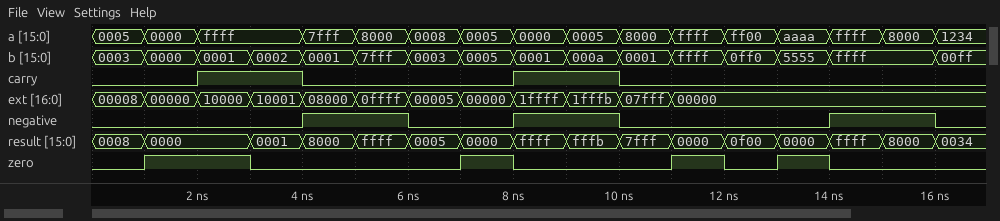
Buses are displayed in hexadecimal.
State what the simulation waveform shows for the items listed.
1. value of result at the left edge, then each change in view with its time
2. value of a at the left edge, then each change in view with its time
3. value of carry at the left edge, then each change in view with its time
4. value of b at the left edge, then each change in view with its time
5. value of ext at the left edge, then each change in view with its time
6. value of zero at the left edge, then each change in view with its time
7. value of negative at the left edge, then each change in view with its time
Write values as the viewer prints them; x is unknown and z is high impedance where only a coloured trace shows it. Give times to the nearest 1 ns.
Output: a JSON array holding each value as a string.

["0008, 0000 at 1 ns, 0001 at 3 ns, 8000 at 4 ns, ffff at 5 ns, 0005 at 6 ns, 0000 at 7 ns, ffff at 8 ns, fffb at 9 ns, 7fff at 10 ns, 0000 at 11 ns, 0f00 at 12 ns, 0000 at 13 ns, ffff at 14 ns, 8000 at 15 ns, 0034 at 16 ns", "0005, 0000 at 1 ns, ffff at 2 ns, 7fff at 4 ns, 8000 at 5 ns, 0008 at 6 ns, 0005 at 7 ns, 0000 at 8 ns, 0005 at 9 ns, 8000 at 10 ns, ffff at 11 ns, ff00 at 12 ns, aaaa at 13 ns, ffff at 14 ns, 8000 at 15 ns, 1234 at 16 ns", "0, 1 at 2 ns, 0 at 4 ns, 1 at 8 ns, 0 at 10 ns", "0003, 0000 at 1 ns, 0001 at 2 ns, 0002 at 3 ns, 0001 at 4 ns, 7fff at 5 ns, 0003 at 6 ns, 0005 at 7 ns, 0001 at 8 ns, 000a at 9 ns, 0001 at 10 ns, ffff at 11 ns, 0ff0 at 12 ns, 5555 at 13 ns, ffff at 14 ns, 00ff at 16 ns", "00008, 00000 at 1 ns, 10000 at 2 ns, 10001 at 3 ns, 08000 at 4 ns, 0ffff at 5 ns, 00005 at 6 ns, 00000 at 7 ns, 1ffff at 8 ns, 1fffb at 9 ns, 07fff at 10 ns, 00000 at 11 ns", "0, 1 at 1 ns, 0 at 3 ns, 1 at 7 ns, 0 at 8 ns, 1 at 11 ns, 0 at 12 ns, 1 at 13 ns, 0 at 14 ns", "0, 1 at 4 ns, 0 at 6 ns, 1 at 8 ns, 0 at 10 ns, 1 at 14 ns, 0 at 16 ns"]
